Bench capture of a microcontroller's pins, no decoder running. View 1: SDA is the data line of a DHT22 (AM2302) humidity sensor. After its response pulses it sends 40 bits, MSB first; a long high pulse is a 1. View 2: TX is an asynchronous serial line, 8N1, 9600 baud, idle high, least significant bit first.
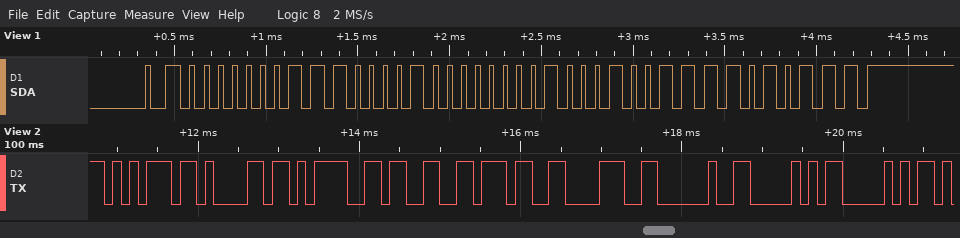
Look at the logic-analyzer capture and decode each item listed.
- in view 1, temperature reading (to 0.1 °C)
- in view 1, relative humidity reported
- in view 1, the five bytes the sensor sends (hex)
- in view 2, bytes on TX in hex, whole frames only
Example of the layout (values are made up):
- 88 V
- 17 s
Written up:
- 27.5 °C
- 45.0 %
- 01 C2 01 13 D7
- 0x75 0x61 0x3D 0x33 0x37 0x38 0x20 0x50 0x50
